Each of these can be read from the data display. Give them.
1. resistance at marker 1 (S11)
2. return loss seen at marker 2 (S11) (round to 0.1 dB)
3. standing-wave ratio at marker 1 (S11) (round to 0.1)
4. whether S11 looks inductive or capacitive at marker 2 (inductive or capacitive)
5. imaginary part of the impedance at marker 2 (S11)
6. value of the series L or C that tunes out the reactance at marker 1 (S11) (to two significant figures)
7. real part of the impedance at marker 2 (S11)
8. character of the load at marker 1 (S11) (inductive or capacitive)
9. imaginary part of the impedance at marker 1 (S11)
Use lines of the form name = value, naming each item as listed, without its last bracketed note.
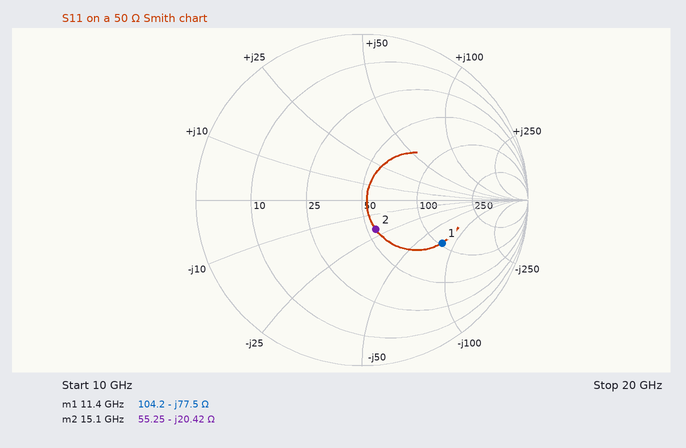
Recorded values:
resistance at marker 1 = 104.2 Ω
return loss seen at marker 2 (S11) = 14.1 dB
standing-wave ratio at marker 1 (S11) = 3.4
whether S11 looks inductive or capacitive at marker 2 = capacitive
imaginary part of the impedance at marker 2 = -20.42 Ω
value of the series L or C that tunes out the reactance at marker 1 (S11) = 1.1 nH
real part of the impedance at marker 2 = 55.25 Ω
character of the load at marker 1 (S11) = capacitive
imaginary part of the impedance at marker 1 = -77.5 Ω
